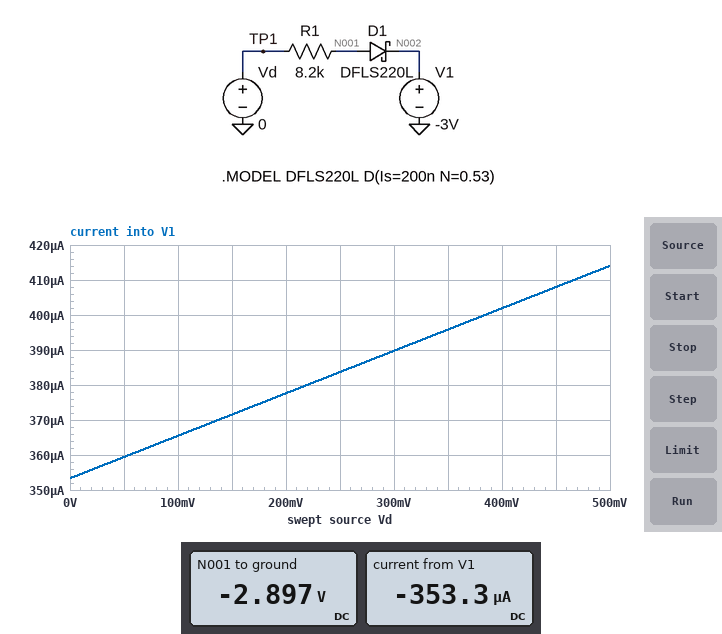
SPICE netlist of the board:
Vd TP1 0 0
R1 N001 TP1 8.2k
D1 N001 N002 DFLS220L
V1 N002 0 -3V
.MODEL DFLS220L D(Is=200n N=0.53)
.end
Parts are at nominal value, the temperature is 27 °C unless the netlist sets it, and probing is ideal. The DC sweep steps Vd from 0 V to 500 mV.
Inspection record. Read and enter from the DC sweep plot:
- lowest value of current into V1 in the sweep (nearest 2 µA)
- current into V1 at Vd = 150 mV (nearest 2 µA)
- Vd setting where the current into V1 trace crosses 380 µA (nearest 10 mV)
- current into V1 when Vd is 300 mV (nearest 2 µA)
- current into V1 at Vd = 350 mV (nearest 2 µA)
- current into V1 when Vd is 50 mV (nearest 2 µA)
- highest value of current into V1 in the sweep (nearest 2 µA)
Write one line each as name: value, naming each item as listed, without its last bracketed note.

lowest value of current into V1 in the sweep: 354 µA
current into V1 at Vd = 150 mV: 372 µA
Vd setting where the current into V1 trace crosses 380 µA: 220 mV
current into V1 when Vd is 300 mV: 390 µA
current into V1 at Vd = 350 mV: 396 µA
current into V1 when Vd is 50 mV: 360 µA
highest value of current into V1 in the sweep: 414 µA
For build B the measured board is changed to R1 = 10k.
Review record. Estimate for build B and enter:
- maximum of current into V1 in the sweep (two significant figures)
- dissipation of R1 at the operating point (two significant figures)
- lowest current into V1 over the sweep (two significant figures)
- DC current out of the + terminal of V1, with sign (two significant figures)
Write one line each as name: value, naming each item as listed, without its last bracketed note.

maximum of current into V1 in the sweep: 340 µA
dissipation of R1 at the operating point: 840 µW
lowest current into V1 over the sweep: 290 µA
DC current out of the + terminal of V1, with sign: -290 µA
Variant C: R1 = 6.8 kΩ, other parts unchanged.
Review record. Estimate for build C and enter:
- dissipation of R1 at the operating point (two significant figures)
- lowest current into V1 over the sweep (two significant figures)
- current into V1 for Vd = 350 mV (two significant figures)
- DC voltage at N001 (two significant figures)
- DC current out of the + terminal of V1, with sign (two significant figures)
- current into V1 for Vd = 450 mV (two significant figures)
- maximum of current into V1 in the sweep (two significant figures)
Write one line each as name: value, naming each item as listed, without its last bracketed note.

dissipation of R1 at the operating point: 1.2 mW
lowest current into V1 over the sweep: 430 µA
current into V1 for Vd = 350 mV: 480 µA
DC voltage at N001: -2.9 V
DC current out of the + terminal of V1, with sign: -430 µA
current into V1 for Vd = 450 mV: 490 µA
maximum of current into V1 in the sweep: 500 µA
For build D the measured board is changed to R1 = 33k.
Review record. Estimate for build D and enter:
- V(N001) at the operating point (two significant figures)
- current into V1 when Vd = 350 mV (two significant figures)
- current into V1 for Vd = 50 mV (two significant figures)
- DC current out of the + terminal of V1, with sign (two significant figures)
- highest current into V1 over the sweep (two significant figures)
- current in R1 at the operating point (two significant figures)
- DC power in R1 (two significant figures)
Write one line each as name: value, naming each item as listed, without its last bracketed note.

V(N001) at the operating point: -2.9 V
current into V1 when Vd = 350 mV: 99 µA
current into V1 for Vd = 50 mV: 90 µA
DC current out of the + terminal of V1, with sign: -88 µA
highest current into V1 over the sweep: 100 µA
current in R1 at the operating point: 88 µA
DC power in R1: 260 µW
